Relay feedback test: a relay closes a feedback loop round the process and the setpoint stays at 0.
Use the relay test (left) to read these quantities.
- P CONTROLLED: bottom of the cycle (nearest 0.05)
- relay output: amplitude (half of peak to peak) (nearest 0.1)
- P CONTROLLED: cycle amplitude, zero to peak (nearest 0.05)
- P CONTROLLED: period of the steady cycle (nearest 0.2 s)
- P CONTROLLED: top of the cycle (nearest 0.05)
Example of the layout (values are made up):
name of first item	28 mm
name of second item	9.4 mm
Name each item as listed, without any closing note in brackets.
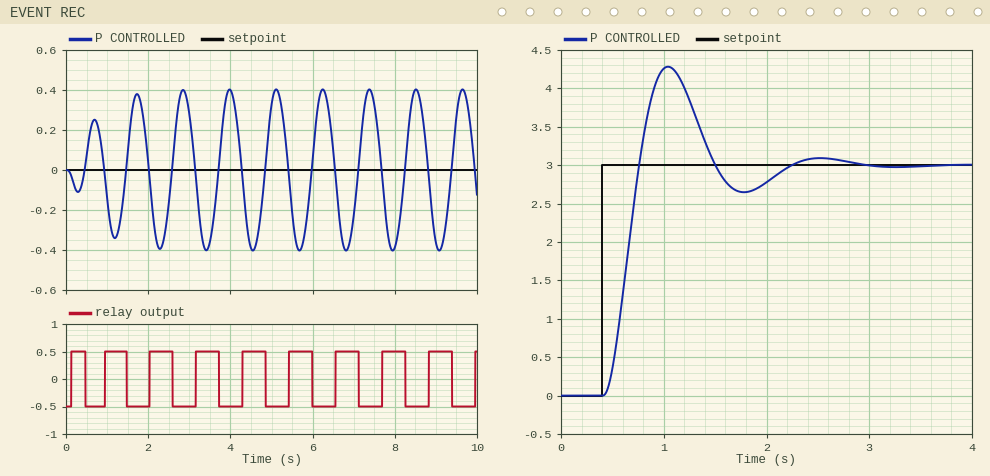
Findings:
P CONTROLLED: bottom of the cycle	-0.40
relay output: amplitude (half of peak to peak)	0.5
P CONTROLLED: cycle amplitude, zero to peak	0.40
P CONTROLLED: period of the steady cycle	1.2 s
P CONTROLLED: top of the cycle	0.40
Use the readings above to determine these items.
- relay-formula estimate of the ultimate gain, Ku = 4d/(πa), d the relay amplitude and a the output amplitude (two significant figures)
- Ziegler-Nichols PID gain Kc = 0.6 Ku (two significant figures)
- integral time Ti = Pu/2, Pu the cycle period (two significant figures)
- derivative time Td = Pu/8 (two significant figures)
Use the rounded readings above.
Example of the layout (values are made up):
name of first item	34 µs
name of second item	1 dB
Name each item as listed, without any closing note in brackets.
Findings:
relay-formula estimate of the ultimate gain, Ku = 4d/(πa), d the relay amplitude and a the output amplitude	1.6
Ziegler-Nichols PID gain Kc = 0.6 Ku	0.96
integral time Ti = Pu/2, Pu the cycle period	0.60 s
derivative time Td = Pu/8	0.15 s
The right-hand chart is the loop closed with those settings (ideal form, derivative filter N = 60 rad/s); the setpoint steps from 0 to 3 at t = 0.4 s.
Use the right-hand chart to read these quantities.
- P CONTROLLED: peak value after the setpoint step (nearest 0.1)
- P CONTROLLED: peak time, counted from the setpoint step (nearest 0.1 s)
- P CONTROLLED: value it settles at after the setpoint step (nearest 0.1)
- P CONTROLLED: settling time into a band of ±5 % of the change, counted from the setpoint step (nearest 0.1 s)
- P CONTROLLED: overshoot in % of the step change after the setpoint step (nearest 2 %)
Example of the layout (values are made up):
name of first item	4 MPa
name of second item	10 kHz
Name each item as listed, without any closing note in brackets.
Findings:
P CONTROLLED: peak value after the setpoint step	4.3
P CONTROLLED: peak time, counted from the setpoint step	0.6 s
P CONTROLLED: value it settles at after the setpoint step	3.0
P CONTROLLED: settling time into a band of ±5 % of the change, counted from the setpoint step	1.7 s
P CONTROLLED: overshoot in % of the step change after the setpoint step	42 %
